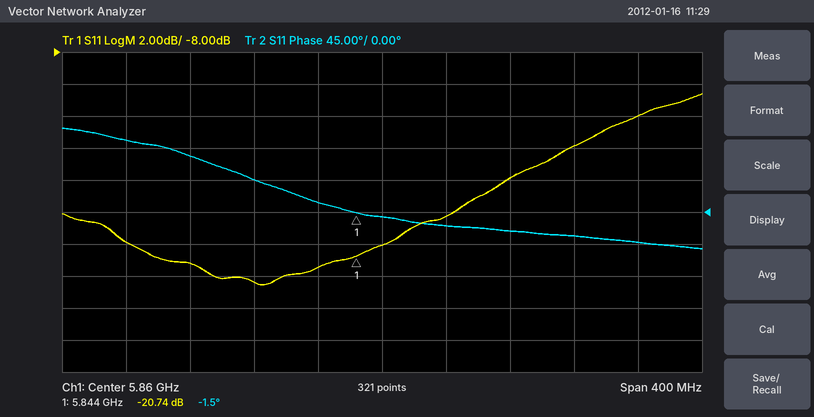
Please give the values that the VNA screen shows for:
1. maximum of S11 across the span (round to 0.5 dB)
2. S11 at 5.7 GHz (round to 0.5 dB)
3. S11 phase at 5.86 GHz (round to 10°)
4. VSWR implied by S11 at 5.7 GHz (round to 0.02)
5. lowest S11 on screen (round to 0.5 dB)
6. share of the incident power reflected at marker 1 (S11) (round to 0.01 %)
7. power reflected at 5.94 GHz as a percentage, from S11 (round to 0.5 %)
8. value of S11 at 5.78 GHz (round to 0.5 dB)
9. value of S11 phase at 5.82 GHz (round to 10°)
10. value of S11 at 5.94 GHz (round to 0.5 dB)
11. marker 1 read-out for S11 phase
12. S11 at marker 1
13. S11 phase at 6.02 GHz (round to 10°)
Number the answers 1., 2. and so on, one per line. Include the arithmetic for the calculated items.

1. -10.5 dB
2. -20.0 dB
3. -10°
4. |Γ| = 10^(-20/20) = 0.1000; VSWR = (1 + 0.1000)/(1 − 0.1000) ≈ 1.22
5. -22.5 dB
6. 10^(-20.74/10) ≈ 0.84 %
7. 10^(-16/10) ≈ 2.5 %
8. -22.5 dB
9. 10°
10. -16.0 dB
11. -1.5°
12. -20.74 dB
13. -40°
